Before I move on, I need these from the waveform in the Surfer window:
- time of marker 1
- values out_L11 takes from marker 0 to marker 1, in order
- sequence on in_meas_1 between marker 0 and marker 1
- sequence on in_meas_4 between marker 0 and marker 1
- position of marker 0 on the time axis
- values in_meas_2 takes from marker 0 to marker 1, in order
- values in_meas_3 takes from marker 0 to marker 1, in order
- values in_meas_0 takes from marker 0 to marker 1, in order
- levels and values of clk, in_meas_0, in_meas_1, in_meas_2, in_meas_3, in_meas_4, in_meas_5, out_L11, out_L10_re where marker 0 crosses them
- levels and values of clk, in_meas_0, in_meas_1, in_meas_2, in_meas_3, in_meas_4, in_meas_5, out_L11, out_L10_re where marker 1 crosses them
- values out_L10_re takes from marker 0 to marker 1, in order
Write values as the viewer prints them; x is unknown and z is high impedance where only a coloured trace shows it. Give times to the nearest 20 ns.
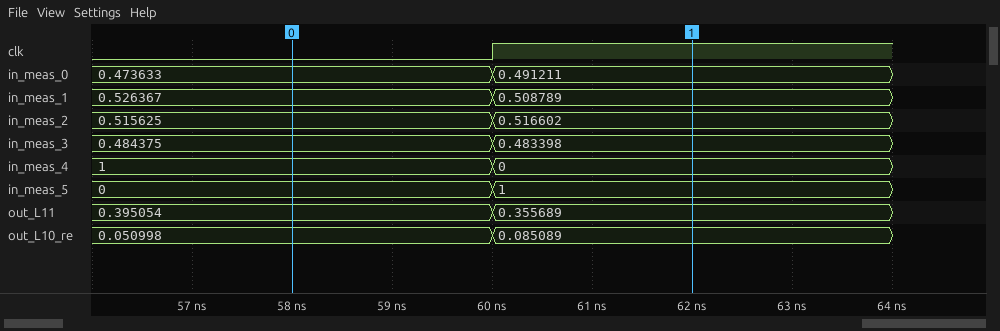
60 ns
0.395054, 0.355689
0.526367, 0.508789
1, 0
60 ns
0.515625, 0.516602
0.484375, 0.483398
0.473633, 0.491211
clk=0, in_meas_0=0.473633, in_meas_1=0.526367, in_meas_2=0.515625, in_meas_3=0.484375, in_meas_4=1, in_meas_5=0, out_L11=0.395054, out_L10_re=0.050998
clk=1, in_meas_0=0.491211, in_meas_1=0.508789, in_meas_2=0.516602, in_meas_3=0.483398, in_meas_4=0, in_meas_5=1, out_L11=0.355689, out_L10_re=0.085089
0.050998, 0.085089
